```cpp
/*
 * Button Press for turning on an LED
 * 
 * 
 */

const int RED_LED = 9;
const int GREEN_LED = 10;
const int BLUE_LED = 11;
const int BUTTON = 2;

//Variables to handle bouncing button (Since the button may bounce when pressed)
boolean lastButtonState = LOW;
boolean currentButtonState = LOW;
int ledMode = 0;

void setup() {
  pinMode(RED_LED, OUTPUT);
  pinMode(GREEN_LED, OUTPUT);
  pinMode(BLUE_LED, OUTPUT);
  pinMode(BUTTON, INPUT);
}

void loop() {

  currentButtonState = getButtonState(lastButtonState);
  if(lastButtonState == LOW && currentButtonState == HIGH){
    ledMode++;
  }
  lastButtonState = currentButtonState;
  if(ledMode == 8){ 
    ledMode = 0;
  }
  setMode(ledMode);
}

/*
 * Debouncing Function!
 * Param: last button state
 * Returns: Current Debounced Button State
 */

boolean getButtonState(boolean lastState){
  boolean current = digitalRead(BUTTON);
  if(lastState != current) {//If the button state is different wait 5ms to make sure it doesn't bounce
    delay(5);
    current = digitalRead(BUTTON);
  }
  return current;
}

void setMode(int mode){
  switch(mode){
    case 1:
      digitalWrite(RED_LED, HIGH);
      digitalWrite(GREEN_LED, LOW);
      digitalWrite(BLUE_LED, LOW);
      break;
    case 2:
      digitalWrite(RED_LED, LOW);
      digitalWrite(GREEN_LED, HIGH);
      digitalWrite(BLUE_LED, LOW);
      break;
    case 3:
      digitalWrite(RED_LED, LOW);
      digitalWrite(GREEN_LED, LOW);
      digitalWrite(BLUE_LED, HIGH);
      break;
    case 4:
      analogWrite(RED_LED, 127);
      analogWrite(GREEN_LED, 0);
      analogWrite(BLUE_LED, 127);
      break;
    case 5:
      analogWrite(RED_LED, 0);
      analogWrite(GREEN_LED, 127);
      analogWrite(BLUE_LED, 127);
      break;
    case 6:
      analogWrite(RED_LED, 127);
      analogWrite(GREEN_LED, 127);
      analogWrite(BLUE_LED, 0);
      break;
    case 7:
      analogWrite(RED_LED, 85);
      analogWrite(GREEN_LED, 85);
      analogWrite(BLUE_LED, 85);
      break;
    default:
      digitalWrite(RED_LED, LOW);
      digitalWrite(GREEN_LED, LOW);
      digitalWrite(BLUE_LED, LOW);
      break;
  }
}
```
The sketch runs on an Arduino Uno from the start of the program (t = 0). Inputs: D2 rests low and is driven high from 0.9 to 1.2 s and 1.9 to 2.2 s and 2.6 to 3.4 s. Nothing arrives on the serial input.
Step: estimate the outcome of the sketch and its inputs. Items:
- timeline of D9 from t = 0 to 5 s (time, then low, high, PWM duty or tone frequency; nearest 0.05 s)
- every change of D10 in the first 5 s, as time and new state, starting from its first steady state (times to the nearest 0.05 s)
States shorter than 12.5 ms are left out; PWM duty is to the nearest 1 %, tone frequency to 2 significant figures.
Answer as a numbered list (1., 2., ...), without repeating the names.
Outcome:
1. 0 s low; 0.9 s high; 1.9 s low
2. 0 s low; 1.9 s high; 2.6 s low
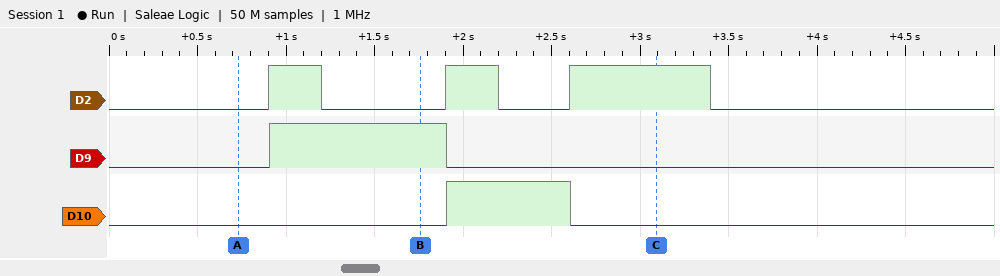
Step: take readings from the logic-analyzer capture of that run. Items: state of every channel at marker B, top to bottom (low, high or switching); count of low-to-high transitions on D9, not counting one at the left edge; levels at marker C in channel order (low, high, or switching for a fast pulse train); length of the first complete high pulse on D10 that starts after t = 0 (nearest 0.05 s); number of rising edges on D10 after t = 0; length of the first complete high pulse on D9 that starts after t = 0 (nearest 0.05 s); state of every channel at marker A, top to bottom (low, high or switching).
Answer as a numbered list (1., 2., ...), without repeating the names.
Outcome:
1. D2 low, D9 high, D10 low
2. 1
3. D2 high, D9 low, D10 low
4. 0.70 s
5. 1
6. 1.00 s
7. D2 low, D9 low, D10 low
